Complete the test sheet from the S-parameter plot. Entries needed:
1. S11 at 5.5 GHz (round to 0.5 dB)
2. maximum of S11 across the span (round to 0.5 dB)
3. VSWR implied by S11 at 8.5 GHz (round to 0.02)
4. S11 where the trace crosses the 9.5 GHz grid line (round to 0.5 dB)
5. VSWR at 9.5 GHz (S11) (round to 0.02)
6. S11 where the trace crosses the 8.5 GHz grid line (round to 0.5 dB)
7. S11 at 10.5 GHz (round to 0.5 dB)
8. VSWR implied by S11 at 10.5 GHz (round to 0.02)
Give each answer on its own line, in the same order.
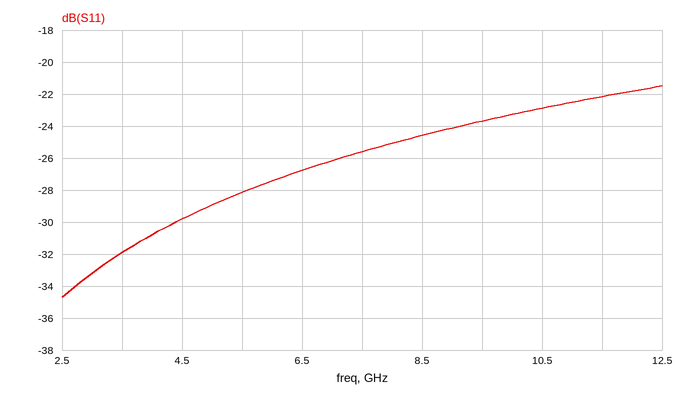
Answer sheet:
-28.0 dB
-21.5 dB
1.12
-23.5 dB
1.14
-24.5 dB
-23.0 dB
1.16
